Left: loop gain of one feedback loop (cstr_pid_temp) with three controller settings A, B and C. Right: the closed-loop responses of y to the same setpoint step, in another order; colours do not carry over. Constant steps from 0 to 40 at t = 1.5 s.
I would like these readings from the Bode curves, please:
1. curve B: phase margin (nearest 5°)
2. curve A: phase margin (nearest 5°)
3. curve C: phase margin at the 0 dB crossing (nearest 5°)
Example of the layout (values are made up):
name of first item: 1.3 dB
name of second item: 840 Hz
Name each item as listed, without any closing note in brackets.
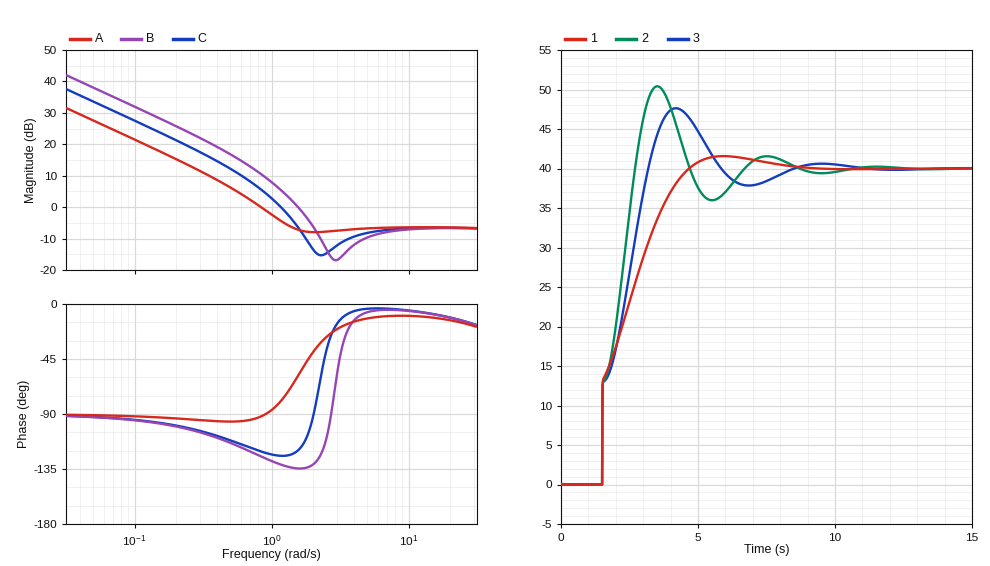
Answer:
curve B: phase margin: 45°
curve A: phase margin: 90°
curve C: phase margin at the 0 dB crossing: 55°
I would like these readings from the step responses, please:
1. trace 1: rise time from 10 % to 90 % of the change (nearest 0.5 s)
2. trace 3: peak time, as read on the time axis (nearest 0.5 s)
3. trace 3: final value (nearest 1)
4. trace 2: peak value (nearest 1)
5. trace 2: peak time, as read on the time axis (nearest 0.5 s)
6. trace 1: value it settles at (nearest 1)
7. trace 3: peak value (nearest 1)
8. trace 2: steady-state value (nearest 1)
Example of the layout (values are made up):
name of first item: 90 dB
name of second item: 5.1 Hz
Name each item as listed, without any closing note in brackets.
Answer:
trace 1: rise time from 10 % to 90 % of the change: 2.5 s
trace 3: peak time, as read on the time axis: 4.0 s
trace 3: final value: 40
trace 2: peak value: 50
trace 2: peak time, as read on the time axis: 3.5 s
trace 1: value it settles at: 40
trace 3: peak value: 48
trace 2: steady-state value: 40
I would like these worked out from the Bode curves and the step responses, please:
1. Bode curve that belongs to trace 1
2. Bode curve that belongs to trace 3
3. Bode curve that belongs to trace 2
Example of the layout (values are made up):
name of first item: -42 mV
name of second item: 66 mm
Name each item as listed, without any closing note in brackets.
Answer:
Bode curve that belongs to trace 1: A
Bode curve that belongs to trace 3: C
Bode curve that belongs to trace 2: B
